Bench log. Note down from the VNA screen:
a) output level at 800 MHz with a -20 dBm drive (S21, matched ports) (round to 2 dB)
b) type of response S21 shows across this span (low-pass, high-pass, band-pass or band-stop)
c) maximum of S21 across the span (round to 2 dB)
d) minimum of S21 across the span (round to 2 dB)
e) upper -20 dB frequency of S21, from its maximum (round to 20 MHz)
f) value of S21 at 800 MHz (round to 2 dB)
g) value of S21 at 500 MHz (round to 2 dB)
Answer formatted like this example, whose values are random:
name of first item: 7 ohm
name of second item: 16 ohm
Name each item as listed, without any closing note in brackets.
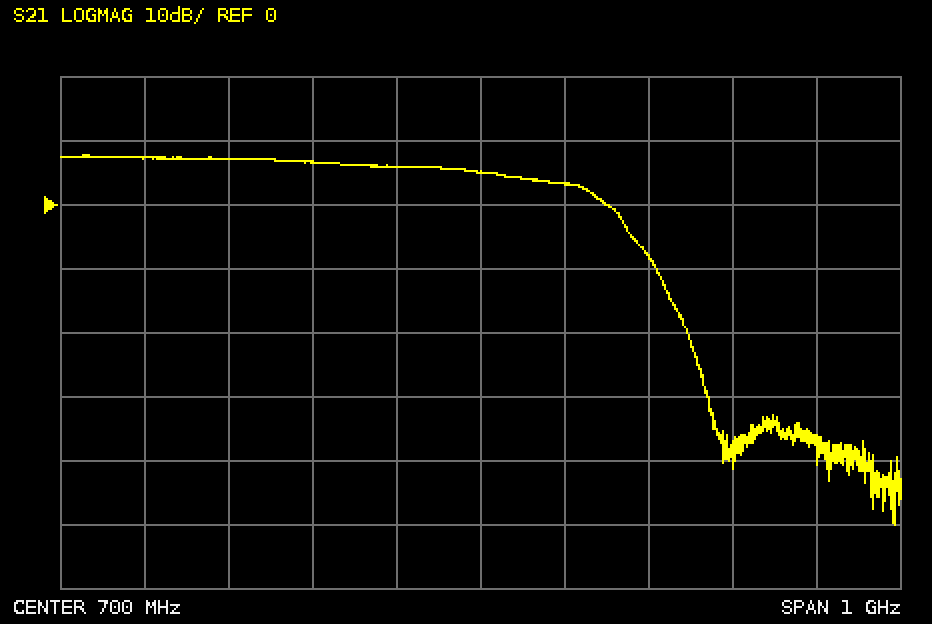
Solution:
output level at 800 MHz with a -20 dBm drive (S21, matched ports): -16 dBm
type of response S21 shows across this span: low-pass
maximum of S21 across the span: 8 dB
minimum of S21 across the span: -50 dB
upper -20 dB frequency of S21, from its maximum: 920 MHz
value of S21 at 800 MHz: 4 dB
value of S21 at 500 MHz: 6 dB
